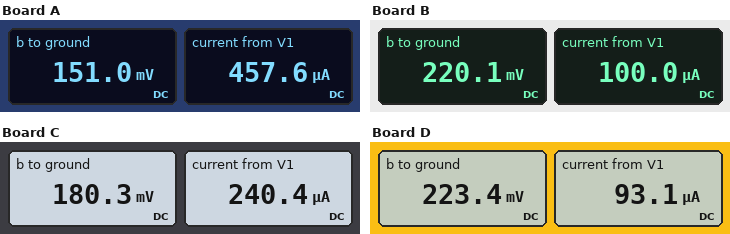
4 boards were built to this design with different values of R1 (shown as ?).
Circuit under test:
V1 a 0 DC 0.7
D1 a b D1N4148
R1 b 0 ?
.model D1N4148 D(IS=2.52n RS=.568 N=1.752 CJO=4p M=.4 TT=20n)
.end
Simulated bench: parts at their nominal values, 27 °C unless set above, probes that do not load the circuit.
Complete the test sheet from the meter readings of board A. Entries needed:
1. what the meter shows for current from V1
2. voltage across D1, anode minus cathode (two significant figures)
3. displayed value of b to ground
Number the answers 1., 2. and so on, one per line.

1. 457.6 µA
2. 550 mV
3. 151.0 mV
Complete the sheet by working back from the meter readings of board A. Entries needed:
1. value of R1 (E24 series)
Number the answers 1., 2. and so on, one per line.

1. 330 Ω
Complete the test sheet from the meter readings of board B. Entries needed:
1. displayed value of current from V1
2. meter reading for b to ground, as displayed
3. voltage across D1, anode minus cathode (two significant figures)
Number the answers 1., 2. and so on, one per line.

1. 100.0 µA
2. 220.1 mV
3. 480 mV
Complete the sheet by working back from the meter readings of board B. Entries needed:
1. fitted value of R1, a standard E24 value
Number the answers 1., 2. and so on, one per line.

1. 2.2 kΩ
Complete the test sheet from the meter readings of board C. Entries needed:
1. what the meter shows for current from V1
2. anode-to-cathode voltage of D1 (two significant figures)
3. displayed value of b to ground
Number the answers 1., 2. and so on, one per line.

1. 240.4 µA
2. 520 mV
3. 180.3 mV
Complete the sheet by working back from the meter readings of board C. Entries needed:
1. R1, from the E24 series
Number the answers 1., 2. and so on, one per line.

1. 750 Ω
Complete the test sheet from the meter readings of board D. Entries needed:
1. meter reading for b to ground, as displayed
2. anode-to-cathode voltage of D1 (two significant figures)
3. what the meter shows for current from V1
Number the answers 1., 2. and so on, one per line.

1. 223.4 mV
2. 480 mV
3. 93.1 µA
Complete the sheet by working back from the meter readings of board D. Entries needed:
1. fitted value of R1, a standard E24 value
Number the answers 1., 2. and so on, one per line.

1. 2.4 kΩ
